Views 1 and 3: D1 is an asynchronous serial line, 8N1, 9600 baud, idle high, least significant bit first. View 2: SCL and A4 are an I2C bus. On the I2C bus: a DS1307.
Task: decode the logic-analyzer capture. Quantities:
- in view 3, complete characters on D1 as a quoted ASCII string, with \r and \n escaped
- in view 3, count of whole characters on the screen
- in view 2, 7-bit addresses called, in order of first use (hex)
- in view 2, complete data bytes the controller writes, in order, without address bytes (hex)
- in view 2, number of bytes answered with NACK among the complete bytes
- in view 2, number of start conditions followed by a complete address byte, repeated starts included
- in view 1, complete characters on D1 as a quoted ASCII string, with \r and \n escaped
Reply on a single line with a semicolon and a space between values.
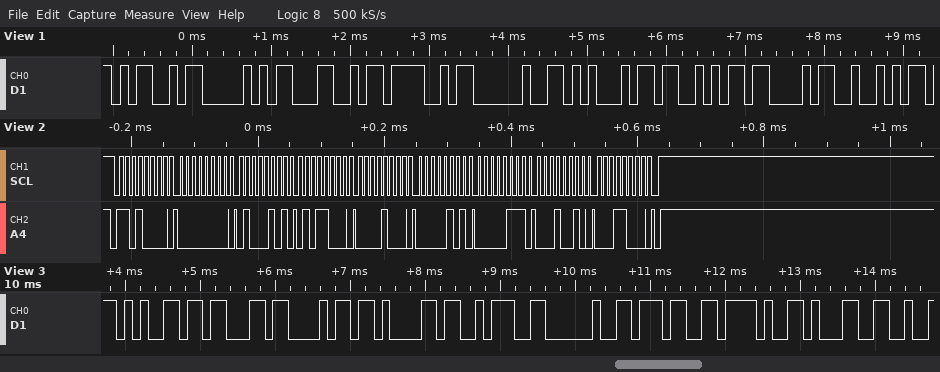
"echa: 7/1"; 9; 0x68; 00 45 58 08 05 07 12 18; 0; 1; "MPLO ESCR"
